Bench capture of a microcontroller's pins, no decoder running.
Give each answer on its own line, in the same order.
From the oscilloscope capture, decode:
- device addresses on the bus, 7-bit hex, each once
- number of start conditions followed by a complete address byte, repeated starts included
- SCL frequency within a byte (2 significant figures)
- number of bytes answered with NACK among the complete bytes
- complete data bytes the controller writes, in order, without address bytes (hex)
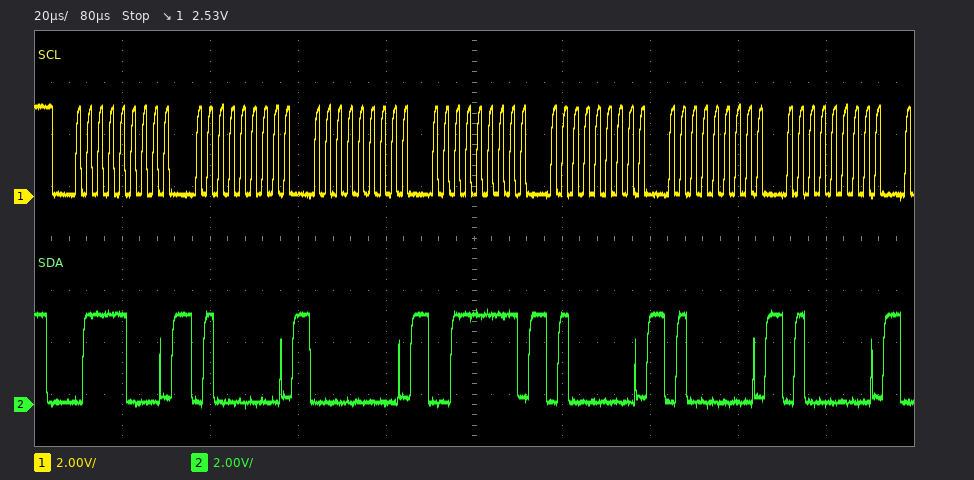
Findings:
0x3C
1
400 kHz
0
40 00 3F 40 40 40
